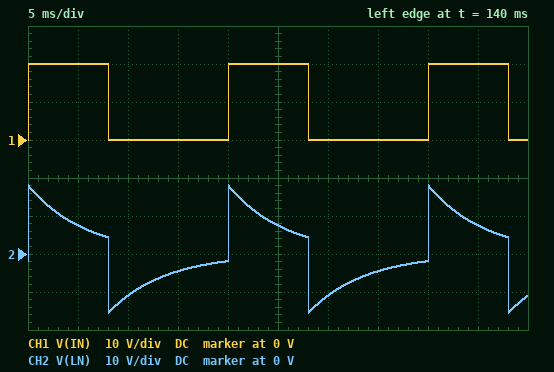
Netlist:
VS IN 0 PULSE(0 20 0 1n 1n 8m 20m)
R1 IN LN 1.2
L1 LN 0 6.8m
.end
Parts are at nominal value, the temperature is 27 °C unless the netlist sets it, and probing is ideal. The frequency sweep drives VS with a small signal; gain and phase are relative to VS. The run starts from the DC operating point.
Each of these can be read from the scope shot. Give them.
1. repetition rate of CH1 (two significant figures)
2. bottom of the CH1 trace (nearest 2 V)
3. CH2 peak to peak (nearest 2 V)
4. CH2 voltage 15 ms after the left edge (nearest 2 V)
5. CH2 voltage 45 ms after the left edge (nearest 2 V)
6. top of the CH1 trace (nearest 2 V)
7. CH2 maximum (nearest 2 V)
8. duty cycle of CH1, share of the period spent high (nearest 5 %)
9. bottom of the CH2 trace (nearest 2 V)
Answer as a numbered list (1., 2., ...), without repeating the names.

1. 50 Hz
2. 0 V
3. 34 V
4. -4 V
5. 8 V
6. 20 V
7. 18 V
8. 40 %
9. -16 V
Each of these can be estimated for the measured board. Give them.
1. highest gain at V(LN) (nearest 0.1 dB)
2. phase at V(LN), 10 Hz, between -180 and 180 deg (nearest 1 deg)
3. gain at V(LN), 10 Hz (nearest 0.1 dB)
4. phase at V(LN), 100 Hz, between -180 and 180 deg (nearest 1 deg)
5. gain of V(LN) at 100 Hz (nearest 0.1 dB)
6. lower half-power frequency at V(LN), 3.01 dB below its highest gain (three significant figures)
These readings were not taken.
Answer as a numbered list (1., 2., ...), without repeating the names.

1. 0 dB
2. 70 deg
3. -9.5 dB
4. 16 deg
5. -0.3 dB
6. 28.1 Hz
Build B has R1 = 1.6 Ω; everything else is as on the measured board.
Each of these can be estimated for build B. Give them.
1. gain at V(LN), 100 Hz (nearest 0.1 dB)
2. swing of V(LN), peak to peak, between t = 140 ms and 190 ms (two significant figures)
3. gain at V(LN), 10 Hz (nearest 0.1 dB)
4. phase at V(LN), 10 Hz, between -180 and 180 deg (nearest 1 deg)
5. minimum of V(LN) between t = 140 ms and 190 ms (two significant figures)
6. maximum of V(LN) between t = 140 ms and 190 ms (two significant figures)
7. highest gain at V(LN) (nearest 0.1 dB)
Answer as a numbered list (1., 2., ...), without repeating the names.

1. -0.6 dB
2. 36 V
3. -11.8 dB
4. 75 deg
5. -17 V
6. 19 V
7. 0 dB
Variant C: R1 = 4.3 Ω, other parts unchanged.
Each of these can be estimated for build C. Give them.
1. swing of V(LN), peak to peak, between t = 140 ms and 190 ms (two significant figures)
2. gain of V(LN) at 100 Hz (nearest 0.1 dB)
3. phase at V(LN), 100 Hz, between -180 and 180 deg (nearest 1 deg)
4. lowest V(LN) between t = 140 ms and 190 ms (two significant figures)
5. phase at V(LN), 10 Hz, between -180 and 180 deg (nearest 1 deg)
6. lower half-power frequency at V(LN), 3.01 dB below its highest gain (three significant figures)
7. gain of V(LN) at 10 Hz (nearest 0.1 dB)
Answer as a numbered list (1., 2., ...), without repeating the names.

1. 40 V
2. -3.0 dB
3. 45 deg
4. -20 V
5. 84 deg
6. 101 Hz
7. -20.1 dB
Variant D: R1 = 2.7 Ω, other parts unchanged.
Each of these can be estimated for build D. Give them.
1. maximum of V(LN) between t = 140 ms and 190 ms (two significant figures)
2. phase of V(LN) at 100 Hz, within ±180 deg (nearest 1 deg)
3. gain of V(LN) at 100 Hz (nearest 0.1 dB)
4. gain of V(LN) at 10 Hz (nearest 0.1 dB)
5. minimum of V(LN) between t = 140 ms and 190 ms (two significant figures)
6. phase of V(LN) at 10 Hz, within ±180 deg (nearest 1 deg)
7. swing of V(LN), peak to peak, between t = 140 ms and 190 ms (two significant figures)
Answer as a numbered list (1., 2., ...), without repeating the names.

1. 20 V
2. 32 deg
3. -1.5 dB
4. -16.1 dB
5. -19 V
6. 81 deg
7. 39 V
